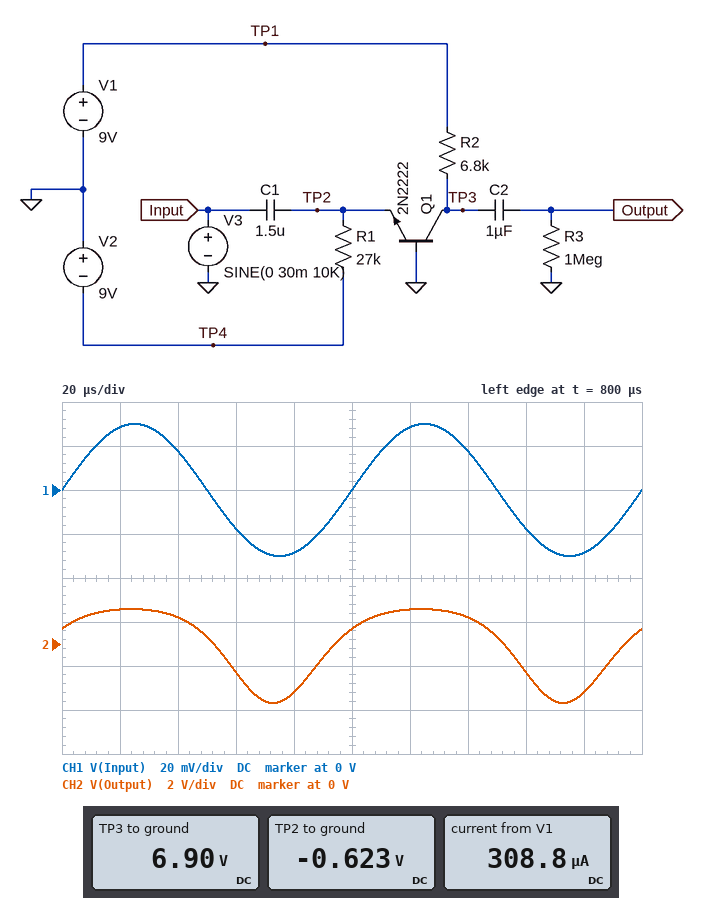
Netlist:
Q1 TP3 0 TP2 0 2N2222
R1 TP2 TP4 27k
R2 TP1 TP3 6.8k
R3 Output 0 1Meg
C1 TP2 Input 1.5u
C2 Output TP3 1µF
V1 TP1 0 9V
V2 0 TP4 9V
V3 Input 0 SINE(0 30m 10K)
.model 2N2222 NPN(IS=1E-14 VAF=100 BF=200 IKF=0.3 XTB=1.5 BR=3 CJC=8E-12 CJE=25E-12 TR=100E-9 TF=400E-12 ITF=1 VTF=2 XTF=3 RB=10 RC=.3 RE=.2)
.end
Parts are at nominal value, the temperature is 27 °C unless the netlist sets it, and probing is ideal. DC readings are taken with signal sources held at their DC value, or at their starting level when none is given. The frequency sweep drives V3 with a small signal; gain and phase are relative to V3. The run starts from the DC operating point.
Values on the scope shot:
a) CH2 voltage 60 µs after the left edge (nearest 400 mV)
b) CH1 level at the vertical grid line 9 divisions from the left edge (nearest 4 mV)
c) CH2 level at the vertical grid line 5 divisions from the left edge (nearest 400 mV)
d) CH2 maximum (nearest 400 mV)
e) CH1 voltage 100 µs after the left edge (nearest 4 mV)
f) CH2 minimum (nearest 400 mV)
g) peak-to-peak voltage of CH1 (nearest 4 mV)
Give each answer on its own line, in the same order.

-1.2 V
-28 mV
800 mV
1.6 V
0 V
-2.8 V
60 mV
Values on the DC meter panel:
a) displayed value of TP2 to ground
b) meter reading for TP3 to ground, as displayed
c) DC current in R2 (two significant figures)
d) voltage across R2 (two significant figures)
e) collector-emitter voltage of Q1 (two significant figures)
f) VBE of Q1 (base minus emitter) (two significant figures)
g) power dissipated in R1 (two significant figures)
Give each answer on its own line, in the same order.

-0.623 V
6.90 V
310 µA
2.1 V
7.5 V
620 mV
2.6 mW
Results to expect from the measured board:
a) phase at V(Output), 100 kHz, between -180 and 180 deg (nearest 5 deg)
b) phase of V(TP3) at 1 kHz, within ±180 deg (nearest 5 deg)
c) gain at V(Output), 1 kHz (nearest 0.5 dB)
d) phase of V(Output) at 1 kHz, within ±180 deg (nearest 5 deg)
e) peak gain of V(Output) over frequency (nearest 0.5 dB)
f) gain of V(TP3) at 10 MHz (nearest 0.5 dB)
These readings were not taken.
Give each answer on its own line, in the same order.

0 deg
50 deg
34.0 dB
50 deg
38.0 dB
32.0 dB
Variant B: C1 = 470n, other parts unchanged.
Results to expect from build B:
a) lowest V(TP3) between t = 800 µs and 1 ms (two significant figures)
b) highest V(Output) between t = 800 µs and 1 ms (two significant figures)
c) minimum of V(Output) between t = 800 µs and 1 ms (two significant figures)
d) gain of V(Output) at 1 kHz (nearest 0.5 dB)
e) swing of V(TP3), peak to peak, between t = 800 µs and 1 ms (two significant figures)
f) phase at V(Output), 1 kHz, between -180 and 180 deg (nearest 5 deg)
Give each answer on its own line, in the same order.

4.4 V
1.5 V
-2.5 V
25.5 dB
4.0 V
75 deg
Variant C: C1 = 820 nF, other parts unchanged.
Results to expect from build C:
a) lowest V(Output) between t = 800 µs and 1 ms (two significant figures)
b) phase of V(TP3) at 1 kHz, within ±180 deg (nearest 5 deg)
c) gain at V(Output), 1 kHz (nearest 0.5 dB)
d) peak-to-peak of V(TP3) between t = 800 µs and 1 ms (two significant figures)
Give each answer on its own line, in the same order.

-2.6 V
65 deg
30.0 dB
4.2 V
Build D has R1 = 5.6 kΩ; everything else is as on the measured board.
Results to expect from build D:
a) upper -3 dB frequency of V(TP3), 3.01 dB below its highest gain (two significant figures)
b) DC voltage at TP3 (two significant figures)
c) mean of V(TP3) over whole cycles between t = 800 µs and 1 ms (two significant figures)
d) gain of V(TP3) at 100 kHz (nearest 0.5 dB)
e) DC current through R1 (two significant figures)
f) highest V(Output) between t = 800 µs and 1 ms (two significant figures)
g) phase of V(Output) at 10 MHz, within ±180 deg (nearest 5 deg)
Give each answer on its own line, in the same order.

1.5 MHz
-610 mV
710 mV
15.0 dB
1.5 mA
4.9 V
-55 deg
